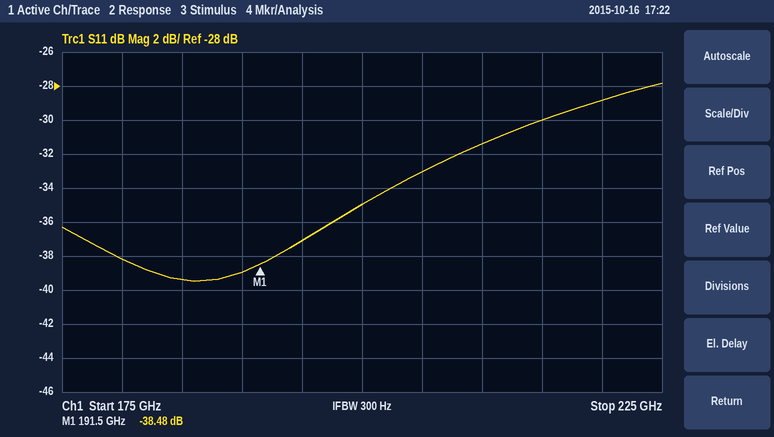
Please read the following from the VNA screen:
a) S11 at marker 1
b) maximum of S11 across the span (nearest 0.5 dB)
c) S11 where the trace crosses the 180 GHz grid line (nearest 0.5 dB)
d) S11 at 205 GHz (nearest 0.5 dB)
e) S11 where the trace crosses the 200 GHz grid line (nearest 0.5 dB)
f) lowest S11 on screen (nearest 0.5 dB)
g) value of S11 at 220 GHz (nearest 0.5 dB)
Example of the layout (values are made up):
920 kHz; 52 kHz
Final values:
-38.48 dB; -28.0 dB; -38.0 dB; -33.0 dB; -35.0 dB; -39.5 dB; -29.0 dB
